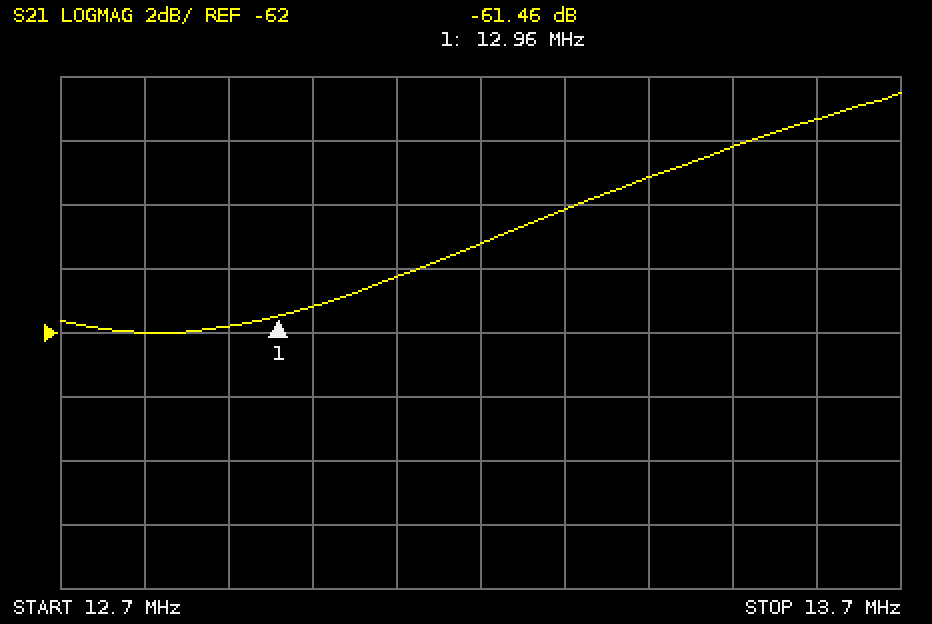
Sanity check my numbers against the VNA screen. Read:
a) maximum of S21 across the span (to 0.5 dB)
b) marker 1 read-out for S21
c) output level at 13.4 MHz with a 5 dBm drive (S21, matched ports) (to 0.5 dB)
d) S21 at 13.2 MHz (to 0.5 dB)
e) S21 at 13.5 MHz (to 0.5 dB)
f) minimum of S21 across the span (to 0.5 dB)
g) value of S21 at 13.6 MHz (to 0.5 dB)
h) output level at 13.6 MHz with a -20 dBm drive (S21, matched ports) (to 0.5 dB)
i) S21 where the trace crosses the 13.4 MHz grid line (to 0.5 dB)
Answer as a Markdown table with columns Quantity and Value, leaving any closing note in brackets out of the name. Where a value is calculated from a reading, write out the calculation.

| Quantity | Value |
|---|---|
| maximum of S21 across the span | -54.5 dB |
| marker 1 read-out for S21 | -61.46 dB |
| output level at 13.4 MHz with a 5 dBm drive (S21, matched ports) | 5 dBm + (-57.0 dB) = -52.0 dBm |
| S21 at 13.2 MHz | -59.0 dB |
| S21 at 13.5 MHz | -56.0 dB |
| minimum of S21 across the span | -62.0 dB |
| value of S21 at 13.6 MHz | -55.5 dB |
| output level at 13.6 MHz with a -20 dBm drive (S21, matched ports) | -20 dBm + (-55.5 dB) = -75.5 dBm |
| S21 where the trace crosses the 13.4 MHz grid line | -57.0 dB |
